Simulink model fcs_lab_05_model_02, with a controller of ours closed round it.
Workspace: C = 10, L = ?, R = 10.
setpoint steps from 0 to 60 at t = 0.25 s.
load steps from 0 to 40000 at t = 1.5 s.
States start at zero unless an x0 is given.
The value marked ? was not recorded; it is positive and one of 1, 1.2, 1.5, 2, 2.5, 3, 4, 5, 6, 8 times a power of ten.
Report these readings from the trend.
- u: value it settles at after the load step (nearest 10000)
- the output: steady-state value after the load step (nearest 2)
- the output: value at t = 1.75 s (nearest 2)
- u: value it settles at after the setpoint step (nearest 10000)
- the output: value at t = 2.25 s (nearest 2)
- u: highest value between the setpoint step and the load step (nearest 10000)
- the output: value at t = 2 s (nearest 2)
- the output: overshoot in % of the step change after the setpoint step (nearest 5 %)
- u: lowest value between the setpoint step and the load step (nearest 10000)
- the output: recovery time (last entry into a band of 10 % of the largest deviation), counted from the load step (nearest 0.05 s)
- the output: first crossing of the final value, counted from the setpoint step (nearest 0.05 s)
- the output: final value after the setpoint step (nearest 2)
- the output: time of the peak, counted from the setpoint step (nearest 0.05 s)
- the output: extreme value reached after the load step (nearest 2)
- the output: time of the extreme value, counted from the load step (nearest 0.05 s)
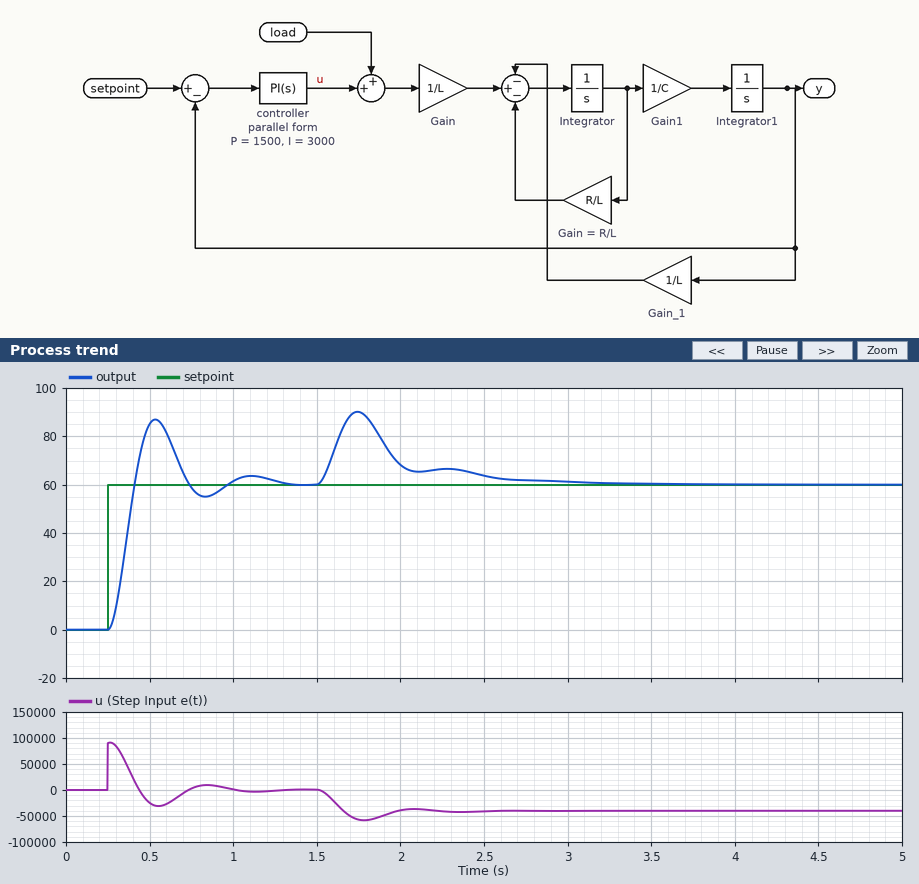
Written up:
-40000
60
90
0
66
90000
68
45 %
-30000
1.05 s
0.15 s
60
0.30 s
90
0.25 s
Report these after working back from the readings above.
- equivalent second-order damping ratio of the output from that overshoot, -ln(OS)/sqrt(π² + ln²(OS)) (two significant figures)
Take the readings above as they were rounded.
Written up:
0.25
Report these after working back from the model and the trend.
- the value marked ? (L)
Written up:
1
